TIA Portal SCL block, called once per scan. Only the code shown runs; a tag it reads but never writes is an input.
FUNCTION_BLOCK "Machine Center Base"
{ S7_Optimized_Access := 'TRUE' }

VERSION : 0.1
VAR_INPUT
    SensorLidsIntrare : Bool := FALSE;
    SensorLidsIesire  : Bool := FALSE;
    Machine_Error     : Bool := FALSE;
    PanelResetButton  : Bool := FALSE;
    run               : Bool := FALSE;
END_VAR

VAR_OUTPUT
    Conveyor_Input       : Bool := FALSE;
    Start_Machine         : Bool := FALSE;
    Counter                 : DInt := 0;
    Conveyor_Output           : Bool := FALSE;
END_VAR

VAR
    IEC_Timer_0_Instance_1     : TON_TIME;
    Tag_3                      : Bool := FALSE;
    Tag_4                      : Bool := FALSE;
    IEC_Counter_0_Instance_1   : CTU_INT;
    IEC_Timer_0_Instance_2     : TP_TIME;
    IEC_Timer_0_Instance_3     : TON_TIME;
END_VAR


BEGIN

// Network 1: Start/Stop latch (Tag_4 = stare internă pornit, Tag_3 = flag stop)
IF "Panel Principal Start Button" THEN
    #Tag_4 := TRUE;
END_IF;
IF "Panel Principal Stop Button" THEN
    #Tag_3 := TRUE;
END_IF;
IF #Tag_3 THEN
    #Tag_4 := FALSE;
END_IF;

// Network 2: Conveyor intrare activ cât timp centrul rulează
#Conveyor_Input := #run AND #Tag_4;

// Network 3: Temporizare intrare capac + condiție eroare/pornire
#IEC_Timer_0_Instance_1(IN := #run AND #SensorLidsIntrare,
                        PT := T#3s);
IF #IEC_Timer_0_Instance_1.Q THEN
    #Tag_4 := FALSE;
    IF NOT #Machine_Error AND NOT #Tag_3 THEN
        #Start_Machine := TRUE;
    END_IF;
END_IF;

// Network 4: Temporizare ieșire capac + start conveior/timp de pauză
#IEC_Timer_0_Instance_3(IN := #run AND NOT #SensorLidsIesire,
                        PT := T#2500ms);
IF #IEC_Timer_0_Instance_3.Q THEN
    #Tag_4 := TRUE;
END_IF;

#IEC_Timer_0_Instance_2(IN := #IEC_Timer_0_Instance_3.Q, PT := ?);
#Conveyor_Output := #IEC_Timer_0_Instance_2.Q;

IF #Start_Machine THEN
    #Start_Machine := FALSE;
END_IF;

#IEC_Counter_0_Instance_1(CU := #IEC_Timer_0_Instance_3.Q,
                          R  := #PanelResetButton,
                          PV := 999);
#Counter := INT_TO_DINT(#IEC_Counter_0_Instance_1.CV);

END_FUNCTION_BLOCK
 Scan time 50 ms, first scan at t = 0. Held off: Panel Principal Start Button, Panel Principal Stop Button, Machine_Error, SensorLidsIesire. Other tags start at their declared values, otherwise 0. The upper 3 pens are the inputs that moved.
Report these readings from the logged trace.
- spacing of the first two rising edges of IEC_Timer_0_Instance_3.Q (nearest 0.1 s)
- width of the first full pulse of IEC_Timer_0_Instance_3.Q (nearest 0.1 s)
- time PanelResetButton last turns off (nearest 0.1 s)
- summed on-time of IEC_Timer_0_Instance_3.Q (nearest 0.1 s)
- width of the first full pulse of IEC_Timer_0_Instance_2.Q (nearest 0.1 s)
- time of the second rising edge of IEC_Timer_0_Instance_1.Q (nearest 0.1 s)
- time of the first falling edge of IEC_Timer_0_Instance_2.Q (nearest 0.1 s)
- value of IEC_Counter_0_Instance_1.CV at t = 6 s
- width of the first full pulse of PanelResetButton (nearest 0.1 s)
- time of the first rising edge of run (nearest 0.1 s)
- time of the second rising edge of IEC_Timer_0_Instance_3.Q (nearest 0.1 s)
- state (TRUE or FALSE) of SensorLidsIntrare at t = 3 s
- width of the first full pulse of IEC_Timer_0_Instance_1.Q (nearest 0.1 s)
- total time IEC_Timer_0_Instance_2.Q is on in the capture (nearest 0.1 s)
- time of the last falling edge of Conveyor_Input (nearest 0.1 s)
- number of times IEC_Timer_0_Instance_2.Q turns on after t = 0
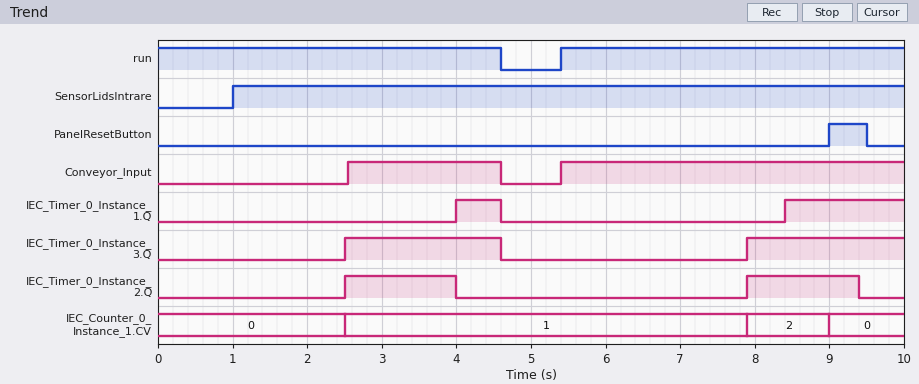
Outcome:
5.4 s
2.1 s
9.5 s
4.2 s
1.5 s
8.4 s
4.0 s
1
0.5 s
5.4 s
7.9 s
TRUE
0.6 s
3.0 s
4.6 s
2
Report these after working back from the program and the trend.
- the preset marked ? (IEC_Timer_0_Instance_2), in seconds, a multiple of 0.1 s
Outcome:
1.5 s
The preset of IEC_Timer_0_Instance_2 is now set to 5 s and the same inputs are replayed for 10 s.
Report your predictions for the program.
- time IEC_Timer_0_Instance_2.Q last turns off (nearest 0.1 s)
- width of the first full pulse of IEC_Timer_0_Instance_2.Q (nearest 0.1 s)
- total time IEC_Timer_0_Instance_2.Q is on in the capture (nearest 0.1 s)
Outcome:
7.5 s
5.0 s
7.1 s
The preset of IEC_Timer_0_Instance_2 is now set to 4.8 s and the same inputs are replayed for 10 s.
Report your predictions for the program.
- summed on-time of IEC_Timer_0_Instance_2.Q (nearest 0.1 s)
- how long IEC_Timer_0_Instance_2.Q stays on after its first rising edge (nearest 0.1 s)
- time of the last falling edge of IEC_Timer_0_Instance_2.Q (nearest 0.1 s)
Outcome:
6.9 s
4.8 s
7.3 s
